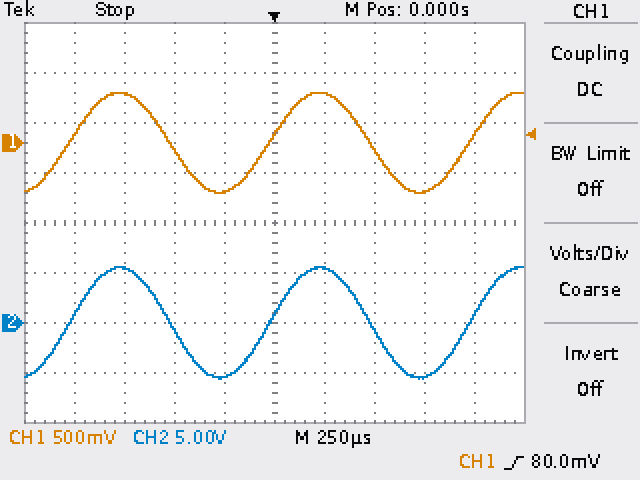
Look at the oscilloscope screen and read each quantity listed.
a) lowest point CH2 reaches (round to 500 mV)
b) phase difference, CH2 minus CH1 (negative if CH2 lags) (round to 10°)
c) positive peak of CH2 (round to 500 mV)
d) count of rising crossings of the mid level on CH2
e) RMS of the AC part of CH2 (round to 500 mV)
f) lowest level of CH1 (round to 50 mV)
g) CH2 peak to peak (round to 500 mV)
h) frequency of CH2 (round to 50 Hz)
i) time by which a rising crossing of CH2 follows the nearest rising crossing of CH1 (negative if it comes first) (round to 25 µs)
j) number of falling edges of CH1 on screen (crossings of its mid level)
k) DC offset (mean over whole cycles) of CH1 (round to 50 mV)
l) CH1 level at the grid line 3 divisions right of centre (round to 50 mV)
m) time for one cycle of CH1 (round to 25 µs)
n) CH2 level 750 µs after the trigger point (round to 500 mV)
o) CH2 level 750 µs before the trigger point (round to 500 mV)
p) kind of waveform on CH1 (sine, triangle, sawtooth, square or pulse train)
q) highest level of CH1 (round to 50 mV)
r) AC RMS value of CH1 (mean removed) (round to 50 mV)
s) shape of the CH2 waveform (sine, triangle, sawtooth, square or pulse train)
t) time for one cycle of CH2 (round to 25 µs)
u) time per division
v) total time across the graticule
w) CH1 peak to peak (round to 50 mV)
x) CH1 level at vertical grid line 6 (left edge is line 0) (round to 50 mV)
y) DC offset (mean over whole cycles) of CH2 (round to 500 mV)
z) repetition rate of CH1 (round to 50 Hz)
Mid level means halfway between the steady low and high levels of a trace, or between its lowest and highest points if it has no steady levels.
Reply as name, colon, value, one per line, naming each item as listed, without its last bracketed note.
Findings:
lowest point CH2 reaches: -5.5 V
phase difference, CH2 minus CH1 (negative if CH2 lags): 0°
positive peak of CH2: 5.5 V
count of rising crossings of the mid level on CH2: 3
RMS of the AC part of CH2: 4.0 V
lowest level of CH1: -500 mV
CH2 peak to peak: 11.0 V
frequency of CH2: 1.00 kHz
time by which a rising crossing of CH2 follows the nearest rising crossing of CH1 (negative if it comes first): 0 µs
number of falling edges of CH1 on screen: 2
DC offset (mean over whole cycles) of CH1: 0 mV
CH1 level at the grid line 3 divisions right of centre: -500 mV
time for one cycle of CH1: 1.000 ms
CH2 level 750 µs after the trigger point: -5.5 V
CH2 level 750 µs before the trigger point: 5.5 V
kind of waveform on CH1: sine
highest level of CH1: 500 mV
AC RMS value of CH1 (mean removed): 350 mV
shape of the CH2 waveform: sine
time for one cycle of CH2: 1.000 ms
time per division: 250 µs
total time across the graticule: 2.5 ms
CH1 peak to peak: 1.00 V
CH1 level at vertical grid line 6 (left edge is line 0): 500 mV
DC offset (mean over whole cycles) of CH2: 0.0 V
repetition rate of CH1: 1.00 kHz
